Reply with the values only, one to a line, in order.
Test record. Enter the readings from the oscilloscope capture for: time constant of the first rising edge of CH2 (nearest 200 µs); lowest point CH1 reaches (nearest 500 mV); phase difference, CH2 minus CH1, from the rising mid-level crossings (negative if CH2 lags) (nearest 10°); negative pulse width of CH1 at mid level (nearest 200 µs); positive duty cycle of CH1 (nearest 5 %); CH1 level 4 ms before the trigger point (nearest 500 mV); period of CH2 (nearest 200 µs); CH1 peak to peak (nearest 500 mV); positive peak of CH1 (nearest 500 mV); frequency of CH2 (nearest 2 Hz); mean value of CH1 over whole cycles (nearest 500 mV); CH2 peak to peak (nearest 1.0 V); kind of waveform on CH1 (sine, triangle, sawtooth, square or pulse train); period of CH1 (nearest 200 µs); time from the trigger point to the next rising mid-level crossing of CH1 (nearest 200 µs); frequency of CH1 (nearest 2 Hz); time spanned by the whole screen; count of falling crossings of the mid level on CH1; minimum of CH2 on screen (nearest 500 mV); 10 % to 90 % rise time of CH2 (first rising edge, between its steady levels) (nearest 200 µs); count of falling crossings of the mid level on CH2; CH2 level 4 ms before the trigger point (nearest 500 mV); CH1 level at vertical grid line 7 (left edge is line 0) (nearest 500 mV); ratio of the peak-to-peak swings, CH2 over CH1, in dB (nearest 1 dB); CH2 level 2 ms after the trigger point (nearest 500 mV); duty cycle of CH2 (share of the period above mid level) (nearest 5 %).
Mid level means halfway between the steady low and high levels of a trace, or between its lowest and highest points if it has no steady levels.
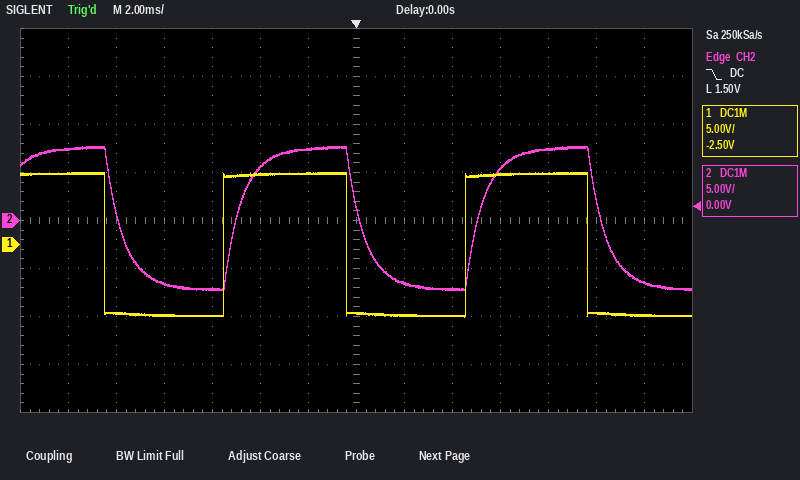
800 µs
-7.5 V
-20°
5.0 ms
50 %
7.5 V
10.0 ms
15.0 V
7.5 V
100 Hz
0.0 V
15.0 V
square
10.0 ms
4.6 ms
100 Hz
28 ms
3
-7.0 V
1.6 ms
3
5.5 V
-7.0 V
0 dB
-6.5 V
50 %
